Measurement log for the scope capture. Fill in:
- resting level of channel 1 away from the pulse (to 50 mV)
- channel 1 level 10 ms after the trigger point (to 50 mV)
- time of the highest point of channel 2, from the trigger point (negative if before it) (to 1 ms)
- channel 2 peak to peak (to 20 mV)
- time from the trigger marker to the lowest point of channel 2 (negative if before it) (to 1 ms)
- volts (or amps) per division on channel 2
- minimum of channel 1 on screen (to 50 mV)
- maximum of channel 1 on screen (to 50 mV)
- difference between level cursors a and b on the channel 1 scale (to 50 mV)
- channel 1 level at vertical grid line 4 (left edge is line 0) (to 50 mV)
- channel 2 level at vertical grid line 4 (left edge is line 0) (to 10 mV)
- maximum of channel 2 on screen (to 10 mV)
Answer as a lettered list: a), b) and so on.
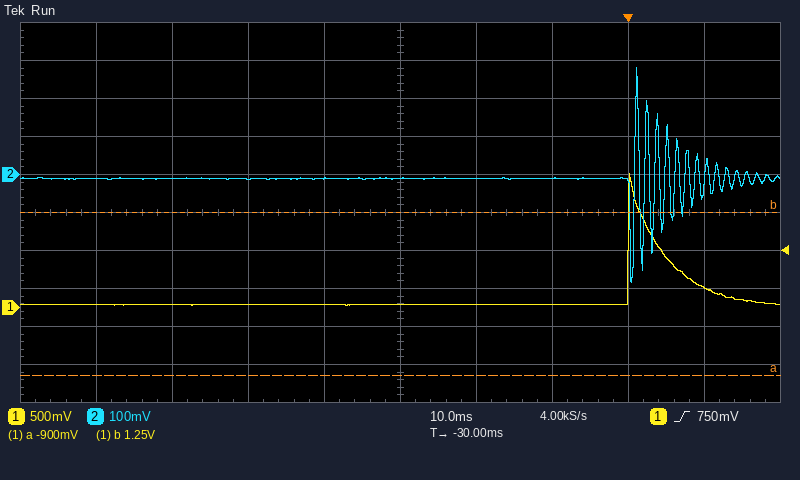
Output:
a) 50 mV
b) 250 mV
c) +1 ms
d) 560 mV
e) 0 ms
f) 100 mV
g) 50 mV
h) 1.75 V
i) 2.15 V
j) 50 mV
k) -10 mV
l) 280 mV
